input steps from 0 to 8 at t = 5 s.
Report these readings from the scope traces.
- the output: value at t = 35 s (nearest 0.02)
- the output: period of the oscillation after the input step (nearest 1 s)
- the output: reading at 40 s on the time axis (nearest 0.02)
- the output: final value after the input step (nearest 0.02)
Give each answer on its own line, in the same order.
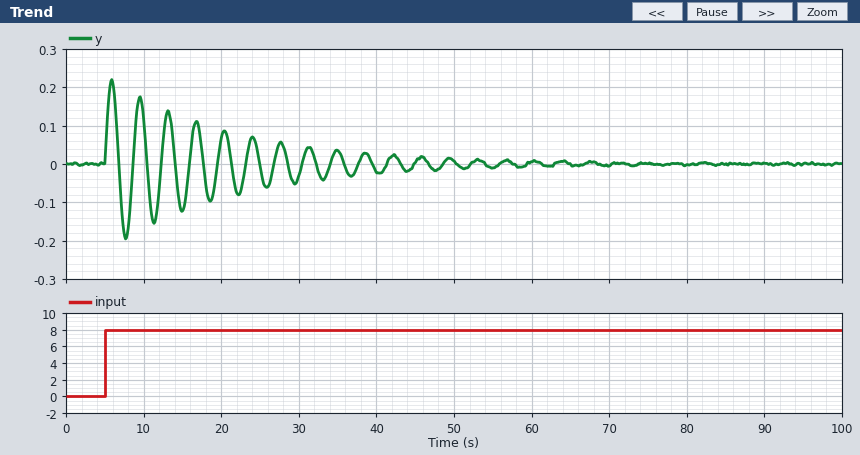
0.04
4 s
-0.02
0.00
